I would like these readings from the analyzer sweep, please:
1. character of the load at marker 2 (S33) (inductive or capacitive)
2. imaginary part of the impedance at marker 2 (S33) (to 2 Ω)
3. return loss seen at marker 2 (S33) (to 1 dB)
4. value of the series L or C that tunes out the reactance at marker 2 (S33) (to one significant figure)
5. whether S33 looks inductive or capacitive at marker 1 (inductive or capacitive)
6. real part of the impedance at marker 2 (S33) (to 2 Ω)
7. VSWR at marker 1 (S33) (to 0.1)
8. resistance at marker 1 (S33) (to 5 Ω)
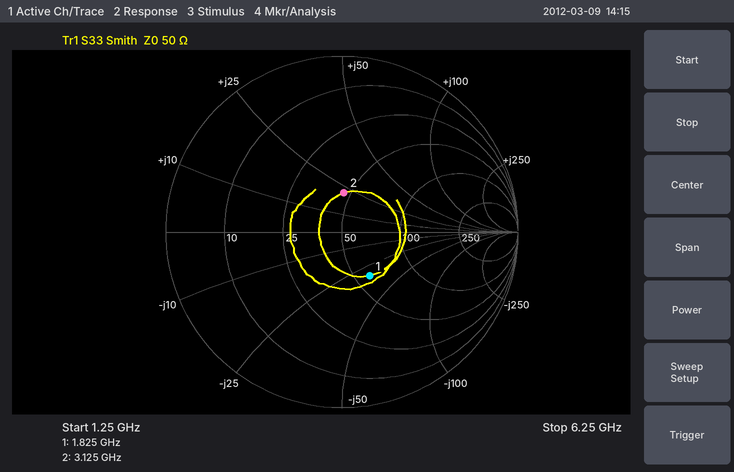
inductive
+22 Ω
13 dB
2 pF
capacitive
46 Ω
1.8
60 Ω
